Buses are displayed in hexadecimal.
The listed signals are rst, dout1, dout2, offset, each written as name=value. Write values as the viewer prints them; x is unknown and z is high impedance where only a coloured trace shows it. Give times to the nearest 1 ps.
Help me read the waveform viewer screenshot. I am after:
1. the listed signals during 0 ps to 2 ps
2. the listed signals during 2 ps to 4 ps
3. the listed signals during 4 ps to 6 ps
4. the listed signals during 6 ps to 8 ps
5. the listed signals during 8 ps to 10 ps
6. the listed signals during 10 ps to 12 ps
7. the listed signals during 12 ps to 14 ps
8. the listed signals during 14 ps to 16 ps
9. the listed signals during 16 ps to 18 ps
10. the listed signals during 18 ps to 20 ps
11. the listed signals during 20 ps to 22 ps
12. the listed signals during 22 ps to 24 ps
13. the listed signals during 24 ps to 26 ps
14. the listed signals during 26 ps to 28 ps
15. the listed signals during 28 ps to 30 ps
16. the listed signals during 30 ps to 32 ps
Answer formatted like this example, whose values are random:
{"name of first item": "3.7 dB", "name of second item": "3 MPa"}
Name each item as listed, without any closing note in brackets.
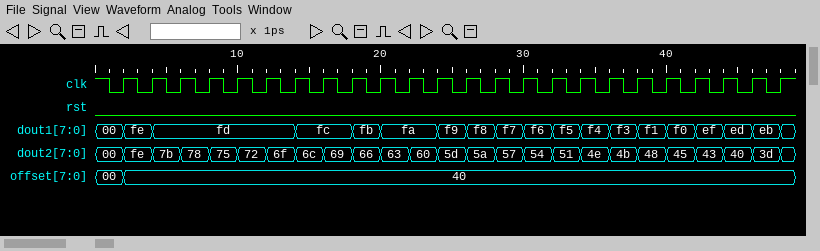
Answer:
{"the listed signals during 0 ps to 2 ps": "rst=0, dout1=00, dout2=00, offset=00", "the listed signals during 2 ps to 4 ps": "rst=0, dout1=fe, dout2=fe, offset=40", "the listed signals during 4 ps to 6 ps": "rst=0, dout1=fd, dout2=7b, offset=40", "the listed signals during 6 ps to 8 ps": "rst=0, dout1=fd, dout2=78, offset=40", "the listed signals during 8 ps to 10 ps": "rst=0, dout1=fd, dout2=75, offset=40", "the listed signals during 10 ps to 12 ps": "rst=0, dout1=fd, dout2=72, offset=40", "the listed signals during 12 ps to 14 ps": "rst=0, dout1=fd, dout2=6f, offset=40", "the listed signals during 14 ps to 16 ps": "rst=0, dout1=fc, dout2=6c, offset=40", "the listed signals during 16 ps to 18 ps": "rst=0, dout1=fc, dout2=69, offset=40", "the listed signals during 18 ps to 20 ps": "rst=0, dout1=fb, dout2=66, offset=40", "the listed signals during 20 ps to 22 ps": "rst=0, dout1=fa, dout2=63, offset=40", "the listed signals during 22 ps to 24 ps": "rst=0, dout1=fa, dout2=60, offset=40", "the listed signals during 24 ps to 26 ps": "rst=0, dout1=f9, dout2=5d, offset=40", "the listed signals during 26 ps to 28 ps": "rst=0, dout1=f8, dout2=5a, offset=40", "the listed signals during 28 ps to 30 ps": "rst=0, dout1=f7, dout2=57, offset=40", "the listed signals during 30 ps to 32 ps": "rst=0, dout1=f6, dout2=54, offset=40"}
